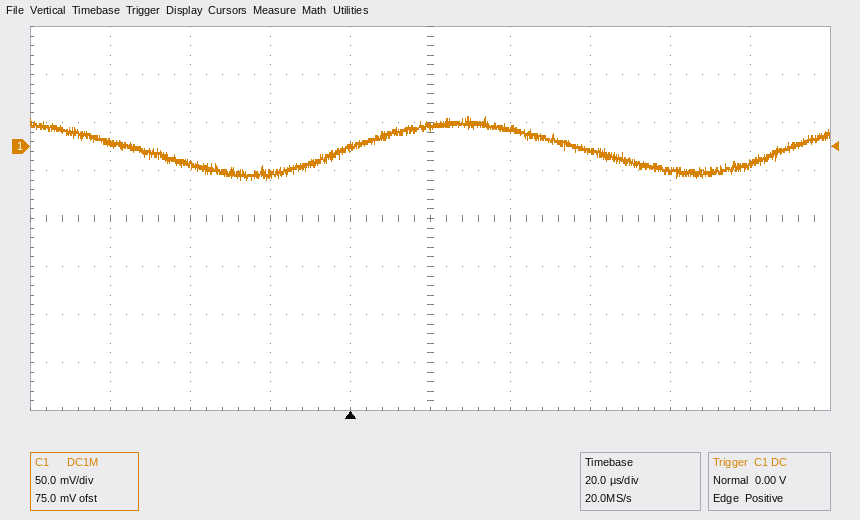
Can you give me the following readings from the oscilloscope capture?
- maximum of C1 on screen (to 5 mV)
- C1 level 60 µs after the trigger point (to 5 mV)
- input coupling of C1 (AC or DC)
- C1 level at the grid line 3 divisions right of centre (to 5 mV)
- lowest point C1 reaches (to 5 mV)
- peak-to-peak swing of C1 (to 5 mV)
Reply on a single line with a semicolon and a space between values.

30 mV; -5 mV; DC; -25 mV; -35 mV; 65 mV
